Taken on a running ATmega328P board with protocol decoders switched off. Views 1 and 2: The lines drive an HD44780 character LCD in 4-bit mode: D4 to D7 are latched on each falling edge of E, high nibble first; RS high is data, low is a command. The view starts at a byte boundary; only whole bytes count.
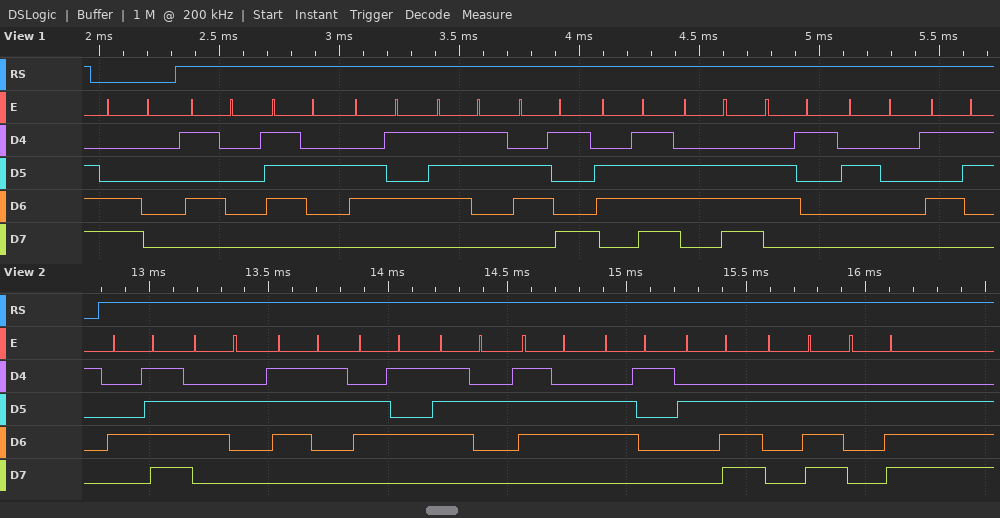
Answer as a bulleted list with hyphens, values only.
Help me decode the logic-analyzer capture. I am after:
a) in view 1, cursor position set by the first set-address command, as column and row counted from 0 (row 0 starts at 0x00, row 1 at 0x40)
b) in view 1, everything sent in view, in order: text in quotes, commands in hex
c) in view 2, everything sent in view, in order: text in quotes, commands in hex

- column 0, row 1
- 0xC0 "Presiona S"
- "Observa..."
